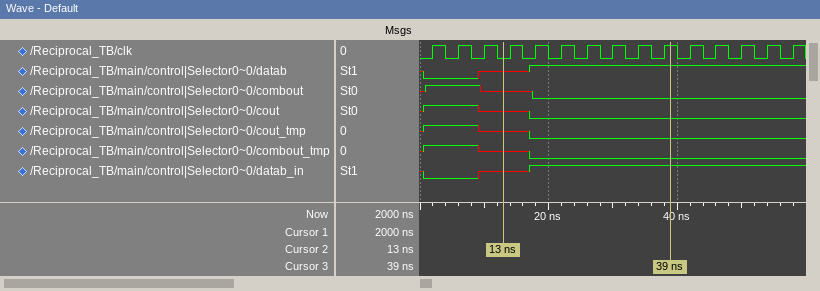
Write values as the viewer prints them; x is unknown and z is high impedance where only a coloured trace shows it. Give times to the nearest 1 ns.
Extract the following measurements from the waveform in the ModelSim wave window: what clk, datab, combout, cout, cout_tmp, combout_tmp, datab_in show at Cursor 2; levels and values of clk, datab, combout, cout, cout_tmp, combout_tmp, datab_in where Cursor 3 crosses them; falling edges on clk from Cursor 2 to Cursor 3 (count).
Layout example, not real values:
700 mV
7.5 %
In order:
clk=0, datab=x, combout=x, cout=x, cout_tmp=x, combout_tmp=x, datab_in=x
clk=1, datab=1, combout=0, cout=0, cout_tmp=0, combout_tmp=0, datab_in=1
6
